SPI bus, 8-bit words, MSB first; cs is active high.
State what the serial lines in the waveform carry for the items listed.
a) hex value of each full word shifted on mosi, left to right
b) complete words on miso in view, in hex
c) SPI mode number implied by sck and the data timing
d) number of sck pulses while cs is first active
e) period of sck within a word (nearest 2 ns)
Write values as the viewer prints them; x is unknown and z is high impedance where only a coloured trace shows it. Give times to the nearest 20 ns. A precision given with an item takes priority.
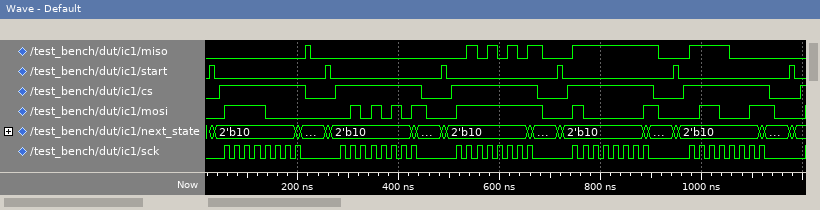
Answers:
F0, 55, FF, 81, 63
00, 00, 55, FF, F0
1
8
20 ns
